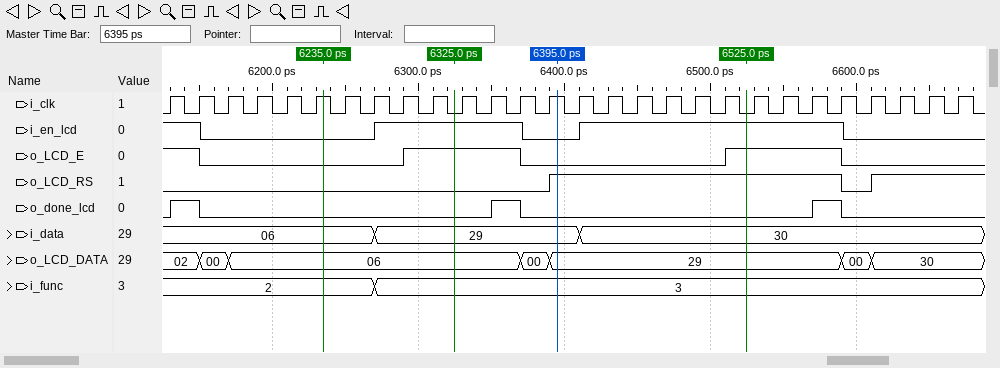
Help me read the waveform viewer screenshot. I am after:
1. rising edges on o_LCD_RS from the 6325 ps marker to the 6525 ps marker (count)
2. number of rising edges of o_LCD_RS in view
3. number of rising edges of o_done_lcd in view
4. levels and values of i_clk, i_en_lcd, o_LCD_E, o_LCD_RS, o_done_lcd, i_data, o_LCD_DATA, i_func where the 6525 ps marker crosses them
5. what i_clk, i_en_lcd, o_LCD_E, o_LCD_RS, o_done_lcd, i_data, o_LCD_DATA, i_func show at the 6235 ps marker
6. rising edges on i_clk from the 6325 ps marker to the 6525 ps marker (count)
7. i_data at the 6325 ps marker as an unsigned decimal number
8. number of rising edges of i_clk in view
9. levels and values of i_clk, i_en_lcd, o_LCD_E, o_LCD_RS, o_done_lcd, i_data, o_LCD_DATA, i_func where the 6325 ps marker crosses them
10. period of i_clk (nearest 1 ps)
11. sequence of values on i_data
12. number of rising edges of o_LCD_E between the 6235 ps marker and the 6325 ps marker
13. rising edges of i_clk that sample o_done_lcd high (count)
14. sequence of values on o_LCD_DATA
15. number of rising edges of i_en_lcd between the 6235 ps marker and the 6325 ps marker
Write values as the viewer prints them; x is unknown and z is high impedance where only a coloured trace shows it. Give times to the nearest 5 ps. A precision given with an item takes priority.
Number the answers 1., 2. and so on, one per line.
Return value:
1. 1
2. 2
3. 3
4. i_clk=0, i_en_lcd=1, o_LCD_E=1, o_LCD_RS=1, o_done_lcd=0, i_data=30, o_LCD_DATA=29, i_func=3
5. i_clk=1, i_en_lcd=0, o_LCD_E=0, o_LCD_RS=0, o_done_lcd=0, i_data=06, o_LCD_DATA=06, i_func=2
6. 10
7. 41
8. 28
9. i_clk=0, i_en_lcd=1, o_LCD_E=1, o_LCD_RS=0, o_done_lcd=0, i_data=29, o_LCD_DATA=06, i_func=3
10. 20 ps
11. 06, 29, 30
12. 1
13. 3
14. 02, 00, 06, 00, 29, 00, 30
15. 1
